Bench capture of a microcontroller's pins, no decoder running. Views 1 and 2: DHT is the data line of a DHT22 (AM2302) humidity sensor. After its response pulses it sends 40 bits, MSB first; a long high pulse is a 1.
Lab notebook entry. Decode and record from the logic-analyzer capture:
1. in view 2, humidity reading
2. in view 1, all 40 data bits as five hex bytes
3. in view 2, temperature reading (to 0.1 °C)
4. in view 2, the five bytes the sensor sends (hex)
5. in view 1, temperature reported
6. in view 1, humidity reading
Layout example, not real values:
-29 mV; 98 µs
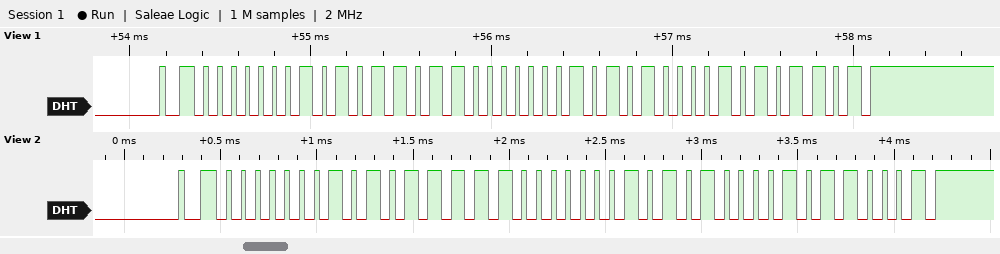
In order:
35.1 %; 01 5B 01 50 AD; 33.6 °C; 01 5F 01 50 B1; 33.6 °C; 34.7 %
